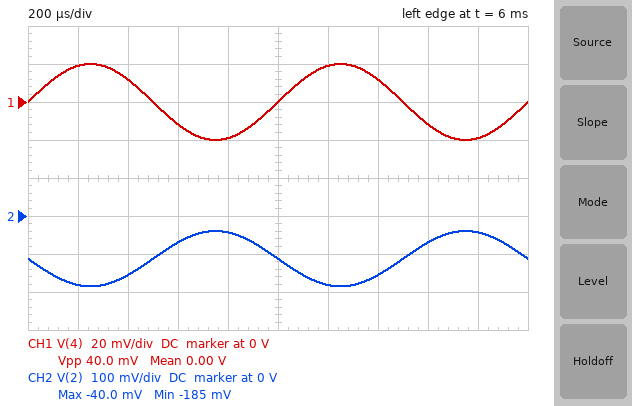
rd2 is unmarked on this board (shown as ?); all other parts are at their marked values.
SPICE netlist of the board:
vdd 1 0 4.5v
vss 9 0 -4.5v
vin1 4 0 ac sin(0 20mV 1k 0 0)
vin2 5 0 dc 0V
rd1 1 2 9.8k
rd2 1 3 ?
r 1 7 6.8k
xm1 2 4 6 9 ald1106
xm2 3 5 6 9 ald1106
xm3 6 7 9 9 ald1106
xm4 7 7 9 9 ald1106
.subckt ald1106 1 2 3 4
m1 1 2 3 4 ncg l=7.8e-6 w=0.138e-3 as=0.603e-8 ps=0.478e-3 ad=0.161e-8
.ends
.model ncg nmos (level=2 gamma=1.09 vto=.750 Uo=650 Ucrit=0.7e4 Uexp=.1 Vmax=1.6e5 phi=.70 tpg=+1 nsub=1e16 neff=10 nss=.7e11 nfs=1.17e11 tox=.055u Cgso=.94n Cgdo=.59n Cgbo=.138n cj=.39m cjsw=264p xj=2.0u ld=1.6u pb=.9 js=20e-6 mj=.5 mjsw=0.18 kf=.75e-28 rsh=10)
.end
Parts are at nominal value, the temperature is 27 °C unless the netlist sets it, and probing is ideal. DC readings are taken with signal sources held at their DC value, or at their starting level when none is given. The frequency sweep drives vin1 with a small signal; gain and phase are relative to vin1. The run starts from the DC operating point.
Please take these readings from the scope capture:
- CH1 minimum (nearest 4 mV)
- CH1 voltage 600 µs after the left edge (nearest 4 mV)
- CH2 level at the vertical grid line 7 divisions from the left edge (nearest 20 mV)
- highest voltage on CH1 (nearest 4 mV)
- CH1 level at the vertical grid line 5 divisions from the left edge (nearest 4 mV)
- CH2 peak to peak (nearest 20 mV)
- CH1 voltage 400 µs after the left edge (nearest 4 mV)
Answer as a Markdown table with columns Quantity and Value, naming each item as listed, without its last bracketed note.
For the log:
| Quantity | Value |
|---|---|
| CH1 minimum | -20 mV |
| CH1 voltage 600 µs after the left edge | -12 mV |
| CH2 level at the vertical grid line 7 divisions from the left edge | -160 mV |
| highest voltage on CH1 | 20 mV |
| CH1 level at the vertical grid line 5 divisions from the left edge | 0 V |
| CH2 peak to peak | 140 mV |
| CH1 voltage 400 µs after the left edge | 12 mV |
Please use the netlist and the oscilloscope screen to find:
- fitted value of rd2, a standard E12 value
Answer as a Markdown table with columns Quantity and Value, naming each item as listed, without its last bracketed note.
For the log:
| Quantity | Value |
|---|---|
| fitted value of rd2, a standard E12 value | 6.8 kΩ |
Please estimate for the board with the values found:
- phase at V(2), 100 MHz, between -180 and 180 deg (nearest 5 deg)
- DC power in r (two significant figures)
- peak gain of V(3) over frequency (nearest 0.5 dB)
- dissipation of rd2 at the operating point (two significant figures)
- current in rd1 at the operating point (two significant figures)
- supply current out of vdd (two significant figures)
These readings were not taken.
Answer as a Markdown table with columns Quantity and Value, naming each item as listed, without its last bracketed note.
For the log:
| Quantity | Value |
|---|---|
| phase at V(2), 100 MHz, between -180 and 180 deg | 125 deg |
| DC power in r | 6.4 mW |
| peak gain of V(3) over frequency | 8.0 dB |
| dissipation of rd2 at the operating point | 1.6 mW |
| current in rd1 at the operating point | 470 µA |
| supply current out of vdd | 1.9 mA |
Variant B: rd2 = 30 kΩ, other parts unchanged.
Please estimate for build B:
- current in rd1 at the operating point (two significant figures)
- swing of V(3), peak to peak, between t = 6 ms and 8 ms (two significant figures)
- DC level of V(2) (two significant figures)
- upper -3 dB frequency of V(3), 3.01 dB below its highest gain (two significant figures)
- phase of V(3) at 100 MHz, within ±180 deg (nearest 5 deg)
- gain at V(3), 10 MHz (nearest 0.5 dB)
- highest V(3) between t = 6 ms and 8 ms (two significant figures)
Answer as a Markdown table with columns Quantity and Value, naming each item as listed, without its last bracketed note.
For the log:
| Quantity | Value |
|---|---|
| current in rd1 at the operating point | 700 µA |
| swing of V(3), peak to peak, between t = 6 ms and 8 ms | 10 mV |
| DC level of V(2) | -2.4 V |
| upper -3 dB frequency of V(3), 3.01 dB below its highest gain | 20 MHz |
| phase of V(3) at 100 MHz, within ±180 deg | -25 deg |
| gain at V(3), 10 MHz | -15.0 dB |
| highest V(3) between t = 6 ms and 8 ms | -2.8 V |
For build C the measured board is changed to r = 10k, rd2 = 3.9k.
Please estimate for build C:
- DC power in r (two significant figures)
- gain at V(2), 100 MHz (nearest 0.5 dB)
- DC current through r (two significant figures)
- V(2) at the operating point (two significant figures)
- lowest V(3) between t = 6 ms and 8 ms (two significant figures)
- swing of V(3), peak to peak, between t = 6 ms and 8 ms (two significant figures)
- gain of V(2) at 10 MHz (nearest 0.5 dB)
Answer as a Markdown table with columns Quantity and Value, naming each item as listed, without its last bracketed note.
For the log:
| Quantity | Value |
|---|---|
| DC power in r | 4.7 mW |
| gain at V(2), 100 MHz | 7.5 dB |
| DC current through r | 690 µA |
| V(2) at the operating point | 1.2 V |
| lowest V(3) between t = 6 ms and 8 ms | 3.1 V |
| swing of V(3), peak to peak, between t = 6 ms and 8 ms | 51 mV |
| gain of V(2) at 10 MHz | 10.5 dB |
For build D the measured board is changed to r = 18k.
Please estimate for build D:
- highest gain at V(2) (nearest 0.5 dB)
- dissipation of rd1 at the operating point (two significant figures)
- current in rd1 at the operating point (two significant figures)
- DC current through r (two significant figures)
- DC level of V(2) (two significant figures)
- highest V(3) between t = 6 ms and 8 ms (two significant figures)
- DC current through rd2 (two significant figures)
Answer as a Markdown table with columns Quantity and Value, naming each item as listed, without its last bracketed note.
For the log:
| Quantity | Value |
|---|---|
| highest gain at V(2) | 9.0 dB |
| dissipation of rd1 at the operating point | 400 µW |
| current in rd1 at the operating point | 200 µA |
| DC current through r | 400 µA |
| DC level of V(2) | 2.5 V |
| highest V(3) between t = 6 ms and 8 ms | 3.1 V |
| DC current through rd2 | 210 µA |
